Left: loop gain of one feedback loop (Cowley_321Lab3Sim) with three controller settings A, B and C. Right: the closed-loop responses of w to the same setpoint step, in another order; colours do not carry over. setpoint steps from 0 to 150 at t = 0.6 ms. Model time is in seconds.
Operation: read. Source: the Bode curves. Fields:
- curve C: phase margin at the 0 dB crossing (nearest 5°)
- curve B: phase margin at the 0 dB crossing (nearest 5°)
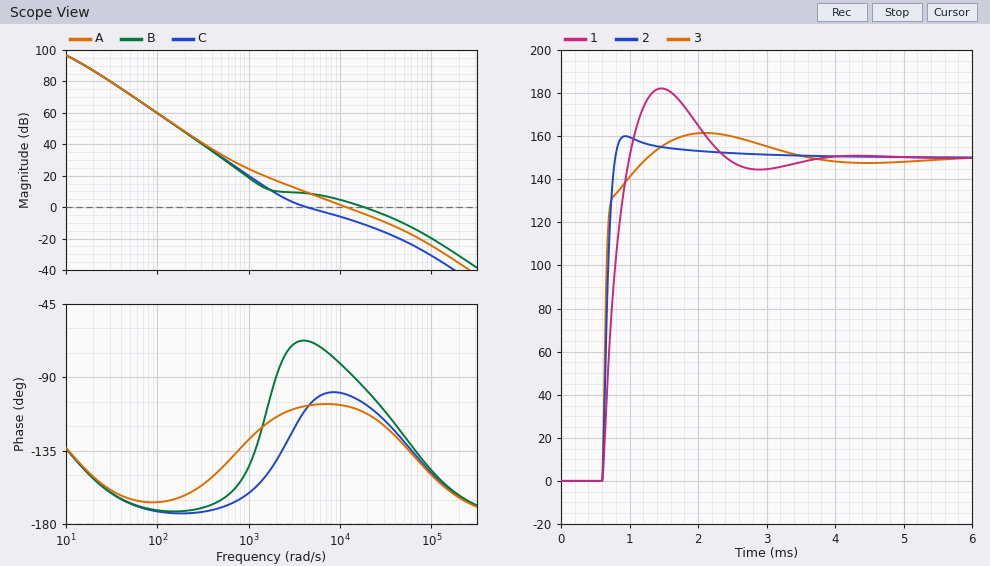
70°
85°
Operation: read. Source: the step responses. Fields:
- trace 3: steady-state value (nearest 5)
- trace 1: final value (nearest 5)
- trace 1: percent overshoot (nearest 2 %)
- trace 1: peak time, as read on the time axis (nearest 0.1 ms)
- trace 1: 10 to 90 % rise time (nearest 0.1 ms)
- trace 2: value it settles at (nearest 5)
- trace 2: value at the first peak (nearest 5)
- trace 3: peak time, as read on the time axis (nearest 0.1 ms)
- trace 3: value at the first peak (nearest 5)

150
150
22 %
1.5 ms
0.3 ms
150
160
2.1 ms
160
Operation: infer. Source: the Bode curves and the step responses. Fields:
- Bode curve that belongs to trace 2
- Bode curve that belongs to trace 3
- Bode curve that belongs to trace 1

A
B
C
